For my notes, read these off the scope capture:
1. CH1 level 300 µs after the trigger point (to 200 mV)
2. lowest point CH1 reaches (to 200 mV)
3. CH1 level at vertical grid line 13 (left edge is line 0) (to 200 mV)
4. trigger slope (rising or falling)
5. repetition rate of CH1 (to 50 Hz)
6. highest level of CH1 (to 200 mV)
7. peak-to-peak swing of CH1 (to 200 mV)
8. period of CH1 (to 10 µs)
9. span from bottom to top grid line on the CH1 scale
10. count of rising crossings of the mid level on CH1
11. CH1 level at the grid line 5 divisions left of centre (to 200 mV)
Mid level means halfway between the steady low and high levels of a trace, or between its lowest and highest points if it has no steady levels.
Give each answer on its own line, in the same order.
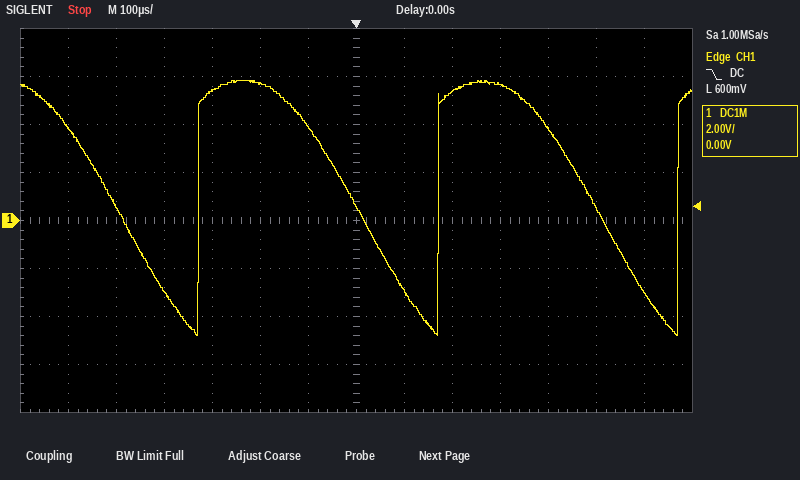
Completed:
5.6 V
-4.8 V
-3.0 V
falling
2.00 kHz
5.8 V
10.6 V
500 µs
16 V
3
600 mV
